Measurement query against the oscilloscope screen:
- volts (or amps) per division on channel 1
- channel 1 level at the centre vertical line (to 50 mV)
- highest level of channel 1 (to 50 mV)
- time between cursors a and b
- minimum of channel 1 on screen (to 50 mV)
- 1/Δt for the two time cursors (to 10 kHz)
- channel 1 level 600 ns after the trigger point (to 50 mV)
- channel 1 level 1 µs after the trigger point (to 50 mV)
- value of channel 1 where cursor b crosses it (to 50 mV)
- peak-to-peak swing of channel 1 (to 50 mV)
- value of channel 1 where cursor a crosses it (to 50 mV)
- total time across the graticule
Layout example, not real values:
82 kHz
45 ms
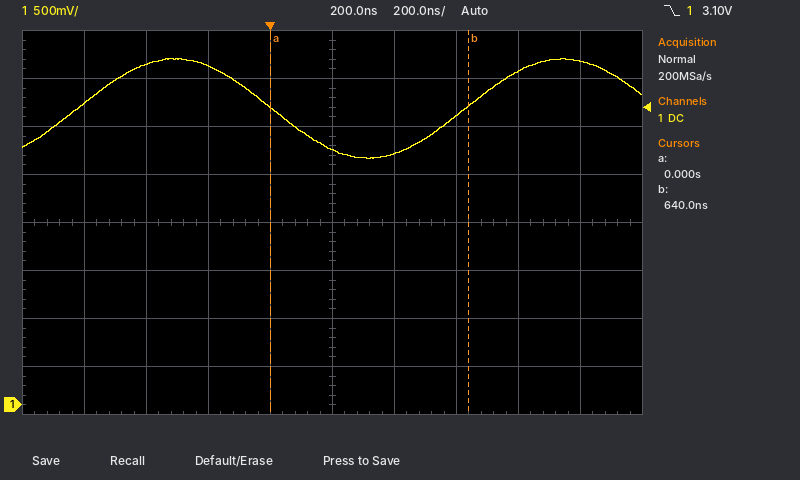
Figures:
500 mV
2.65 V
3.60 V
640 ns
2.55 V
1.56 MHz
3.00 V
3.60 V
3.10 V
1.05 V
3.10 V
2 µs
